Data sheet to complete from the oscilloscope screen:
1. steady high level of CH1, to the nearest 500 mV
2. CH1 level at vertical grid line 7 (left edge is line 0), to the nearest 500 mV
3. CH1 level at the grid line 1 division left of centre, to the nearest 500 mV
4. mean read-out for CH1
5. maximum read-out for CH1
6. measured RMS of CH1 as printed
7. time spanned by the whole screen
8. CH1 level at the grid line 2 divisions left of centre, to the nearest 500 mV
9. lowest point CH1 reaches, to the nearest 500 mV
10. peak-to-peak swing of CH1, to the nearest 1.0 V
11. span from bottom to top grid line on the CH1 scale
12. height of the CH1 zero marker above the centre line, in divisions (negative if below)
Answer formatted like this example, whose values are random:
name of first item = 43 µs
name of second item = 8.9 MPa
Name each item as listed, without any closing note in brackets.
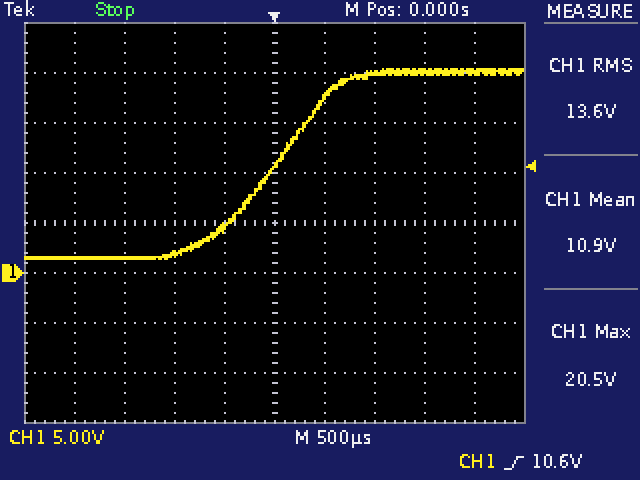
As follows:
steady high level of CH1, to the nearest 500 mV = 20.0 V
CH1 level at vertical grid line 7 (left edge is line 0), to the nearest 500 mV = 20.0 V
CH1 level at the grid line 1 division left of centre, to the nearest 500 mV = 4.5 V
mean read-out for CH1 = 10.9 V
maximum read-out for CH1 = 20.5 V
measured RMS of CH1 as printed = 13.6 V
time spanned by the whole screen = 5 ms
CH1 level at the grid line 2 divisions left of centre, to the nearest 500 mV = 2.0 V
lowest point CH1 reaches, to the nearest 500 mV = 1.5 V
peak-to-peak swing of CH1, to the nearest 1.0 V = 19.0 V
span from bottom to top grid line on the CH1 scale = 40 V
height of the CH1 zero marker above the centre line, in divisions = -1.0 div
